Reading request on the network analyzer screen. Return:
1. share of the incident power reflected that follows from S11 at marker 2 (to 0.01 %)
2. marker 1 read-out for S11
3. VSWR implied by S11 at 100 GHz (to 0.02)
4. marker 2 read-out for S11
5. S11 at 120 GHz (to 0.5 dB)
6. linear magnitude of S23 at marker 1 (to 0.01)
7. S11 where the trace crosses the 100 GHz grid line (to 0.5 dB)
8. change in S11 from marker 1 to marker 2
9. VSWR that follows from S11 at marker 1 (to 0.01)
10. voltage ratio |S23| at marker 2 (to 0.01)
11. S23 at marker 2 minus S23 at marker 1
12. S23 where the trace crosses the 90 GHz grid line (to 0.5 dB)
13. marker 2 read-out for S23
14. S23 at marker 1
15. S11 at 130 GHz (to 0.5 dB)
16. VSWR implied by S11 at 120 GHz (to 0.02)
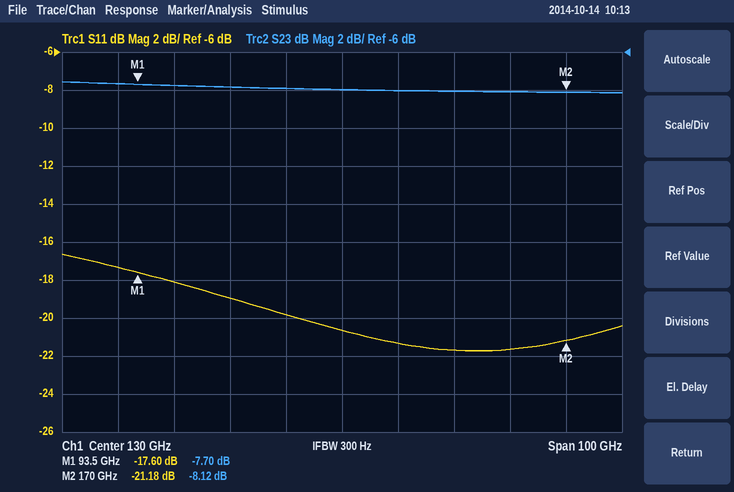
0.76 %
-17.60 dB
1.28
-21.18 dB
-20.0 dB
0.41
-18.0 dB
-3.58 dB
1.30
0.39
-0.42 dB
-7.5 dB
-8.12 dB
-7.70 dB
-20.5 dB
1.22
